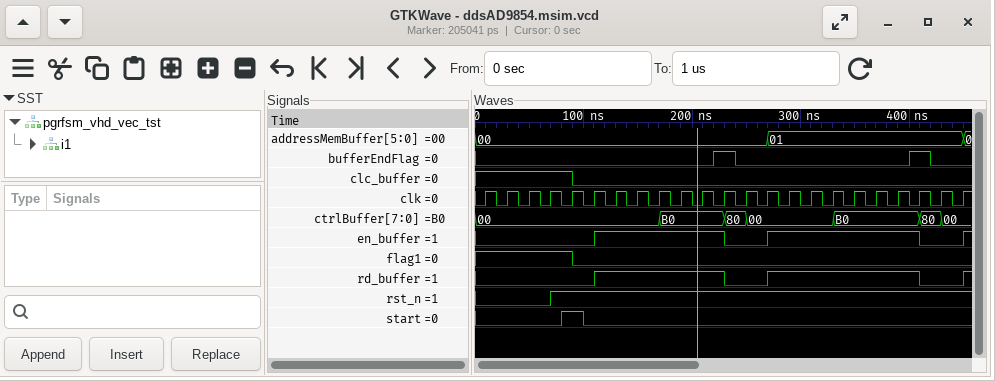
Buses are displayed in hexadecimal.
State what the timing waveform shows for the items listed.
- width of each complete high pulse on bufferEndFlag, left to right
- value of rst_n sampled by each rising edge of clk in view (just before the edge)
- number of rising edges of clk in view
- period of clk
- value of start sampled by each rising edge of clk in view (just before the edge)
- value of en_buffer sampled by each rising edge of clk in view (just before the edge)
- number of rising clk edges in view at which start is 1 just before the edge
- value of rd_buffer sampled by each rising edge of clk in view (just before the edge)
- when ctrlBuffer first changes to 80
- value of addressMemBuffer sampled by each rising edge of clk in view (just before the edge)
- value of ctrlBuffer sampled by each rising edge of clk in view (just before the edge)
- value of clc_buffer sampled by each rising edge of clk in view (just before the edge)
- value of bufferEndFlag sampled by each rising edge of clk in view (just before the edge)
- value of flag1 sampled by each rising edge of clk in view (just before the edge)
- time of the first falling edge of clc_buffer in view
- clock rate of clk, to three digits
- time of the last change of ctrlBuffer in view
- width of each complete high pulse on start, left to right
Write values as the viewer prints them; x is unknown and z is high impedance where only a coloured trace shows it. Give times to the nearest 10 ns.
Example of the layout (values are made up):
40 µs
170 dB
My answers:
20 ns, 20 ns
0 0 0 0 1 1 1 1 1 1 1 1 1 1 1 1 1 1 1 1 1 1 1
23
20 ns
0 0 0 0 1 0 0 0 0 0 0 0 0 0 0 0 0 0 0 0 0 0 0
0 0 0 0 0 0 1 1 1 1 1 1 0 0 1 1 1 1 1 1 1 0 0
1
0 0 0 0 0 0 1 1 1 1 1 1 0 0 1 1 1 1 1 1 1 0 0
230 ns
00, 00, 00, 00, 00, 00, 00, 00, 00, 00, 00, 00, 00, 00, 01, 01, 01, 01, 01, 01, 01, 01, 01
00, 00, 00, 00, 00, 00, 00, 00, 00, B0, B0, B0, 80, 00, 00, 00, 00, B0, B0, B0, B0, 80, 00
1 1 1 1 1 0 0 0 0 0 0 0 0 0 0 0 0 0 0 0 0 0 0
0 0 0 0 0 0 0 0 0 0 0 1 0 0 0 0 0 0 0 0 1 0 0
1 1 1 1 1 0 0 0 0 0 0 0 0 0 0 0 0 0 0 0 0 0 0
90 ns
50.0 MHz
430 ns
20 ns
